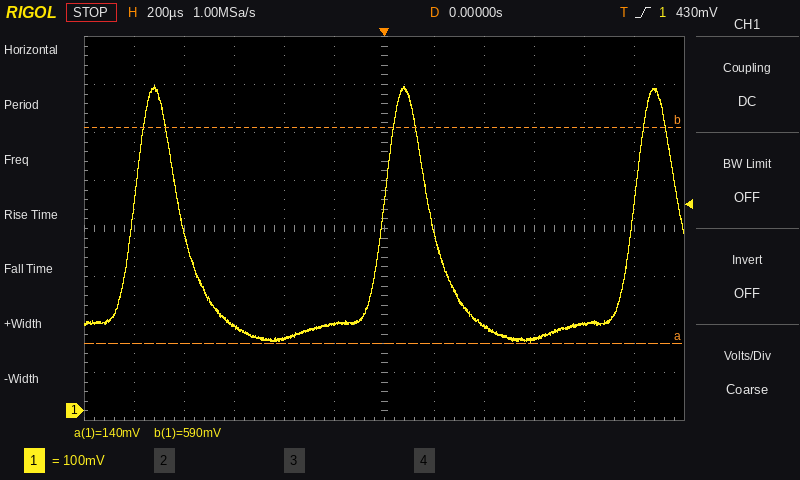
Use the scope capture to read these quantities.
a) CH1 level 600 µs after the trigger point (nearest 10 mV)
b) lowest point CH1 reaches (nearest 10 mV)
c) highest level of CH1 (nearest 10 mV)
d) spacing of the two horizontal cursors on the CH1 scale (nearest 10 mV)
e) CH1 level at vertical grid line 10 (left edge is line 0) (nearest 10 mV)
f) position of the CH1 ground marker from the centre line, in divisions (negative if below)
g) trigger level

150 mV
140 mV
680 mV
450 mV
180 mV
-3.8 div
430 mV
